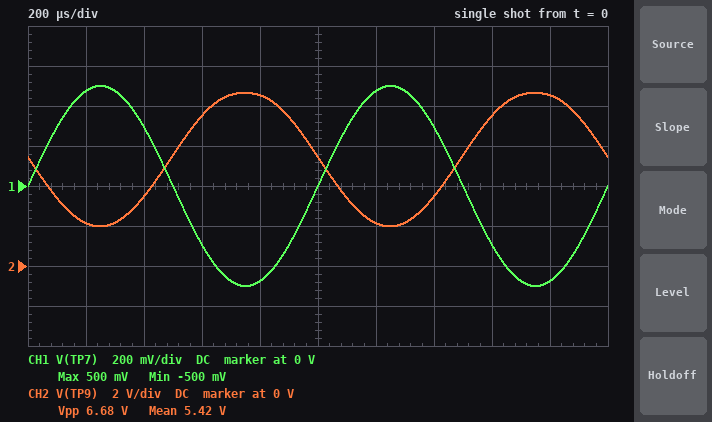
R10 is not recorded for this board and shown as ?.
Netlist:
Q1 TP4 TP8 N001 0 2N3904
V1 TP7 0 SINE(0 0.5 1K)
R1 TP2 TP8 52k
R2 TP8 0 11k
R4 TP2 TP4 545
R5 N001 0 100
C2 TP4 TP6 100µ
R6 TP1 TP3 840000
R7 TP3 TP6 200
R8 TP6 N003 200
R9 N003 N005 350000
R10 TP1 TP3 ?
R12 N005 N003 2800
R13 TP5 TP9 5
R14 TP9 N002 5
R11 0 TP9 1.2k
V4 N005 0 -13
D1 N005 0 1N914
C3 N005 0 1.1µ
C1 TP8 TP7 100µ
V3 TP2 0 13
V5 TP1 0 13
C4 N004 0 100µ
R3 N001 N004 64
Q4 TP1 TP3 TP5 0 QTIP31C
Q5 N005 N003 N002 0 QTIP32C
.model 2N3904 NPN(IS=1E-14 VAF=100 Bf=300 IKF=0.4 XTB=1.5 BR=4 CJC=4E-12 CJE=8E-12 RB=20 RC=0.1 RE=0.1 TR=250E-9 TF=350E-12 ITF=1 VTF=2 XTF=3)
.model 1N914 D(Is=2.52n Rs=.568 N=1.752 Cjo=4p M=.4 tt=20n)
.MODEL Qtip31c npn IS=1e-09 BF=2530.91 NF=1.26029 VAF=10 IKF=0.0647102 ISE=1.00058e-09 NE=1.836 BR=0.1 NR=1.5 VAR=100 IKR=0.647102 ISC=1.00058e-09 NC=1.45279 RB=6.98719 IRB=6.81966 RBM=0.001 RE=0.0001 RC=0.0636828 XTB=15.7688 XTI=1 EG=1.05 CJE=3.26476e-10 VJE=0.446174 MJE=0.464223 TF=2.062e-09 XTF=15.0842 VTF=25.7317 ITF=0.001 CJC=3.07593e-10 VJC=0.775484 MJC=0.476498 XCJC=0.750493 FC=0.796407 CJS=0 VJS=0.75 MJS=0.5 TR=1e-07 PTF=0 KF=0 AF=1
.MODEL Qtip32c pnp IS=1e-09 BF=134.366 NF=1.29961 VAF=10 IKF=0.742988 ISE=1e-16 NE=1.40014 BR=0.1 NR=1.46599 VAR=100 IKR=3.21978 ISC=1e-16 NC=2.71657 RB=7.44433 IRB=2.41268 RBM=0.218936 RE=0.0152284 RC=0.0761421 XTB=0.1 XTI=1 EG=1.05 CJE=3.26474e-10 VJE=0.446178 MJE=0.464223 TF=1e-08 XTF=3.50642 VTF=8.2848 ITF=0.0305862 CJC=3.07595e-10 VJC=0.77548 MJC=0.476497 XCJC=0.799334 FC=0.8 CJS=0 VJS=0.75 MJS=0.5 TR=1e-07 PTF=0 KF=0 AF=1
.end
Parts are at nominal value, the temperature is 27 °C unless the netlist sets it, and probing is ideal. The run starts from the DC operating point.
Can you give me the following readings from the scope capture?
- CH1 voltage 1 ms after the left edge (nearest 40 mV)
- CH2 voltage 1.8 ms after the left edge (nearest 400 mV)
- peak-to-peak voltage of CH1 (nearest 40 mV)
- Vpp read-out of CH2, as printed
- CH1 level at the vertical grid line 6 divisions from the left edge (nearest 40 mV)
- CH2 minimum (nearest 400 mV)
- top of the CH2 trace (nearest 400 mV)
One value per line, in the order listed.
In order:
0 V
8.4 V
1.00 V
6.68 V
480 mV
2.0 V
8.8 V
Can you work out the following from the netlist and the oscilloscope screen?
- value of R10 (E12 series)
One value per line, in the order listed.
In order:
1 kΩ
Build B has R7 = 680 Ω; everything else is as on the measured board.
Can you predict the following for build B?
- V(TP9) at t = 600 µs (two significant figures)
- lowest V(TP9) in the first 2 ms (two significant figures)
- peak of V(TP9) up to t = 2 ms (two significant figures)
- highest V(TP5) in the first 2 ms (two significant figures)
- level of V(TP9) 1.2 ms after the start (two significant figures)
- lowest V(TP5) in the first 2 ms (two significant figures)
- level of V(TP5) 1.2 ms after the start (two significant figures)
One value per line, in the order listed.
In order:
6.7 V
1.6 V
7.8 V
8.7 V
1.7 V
3.6 V
3.7 V
